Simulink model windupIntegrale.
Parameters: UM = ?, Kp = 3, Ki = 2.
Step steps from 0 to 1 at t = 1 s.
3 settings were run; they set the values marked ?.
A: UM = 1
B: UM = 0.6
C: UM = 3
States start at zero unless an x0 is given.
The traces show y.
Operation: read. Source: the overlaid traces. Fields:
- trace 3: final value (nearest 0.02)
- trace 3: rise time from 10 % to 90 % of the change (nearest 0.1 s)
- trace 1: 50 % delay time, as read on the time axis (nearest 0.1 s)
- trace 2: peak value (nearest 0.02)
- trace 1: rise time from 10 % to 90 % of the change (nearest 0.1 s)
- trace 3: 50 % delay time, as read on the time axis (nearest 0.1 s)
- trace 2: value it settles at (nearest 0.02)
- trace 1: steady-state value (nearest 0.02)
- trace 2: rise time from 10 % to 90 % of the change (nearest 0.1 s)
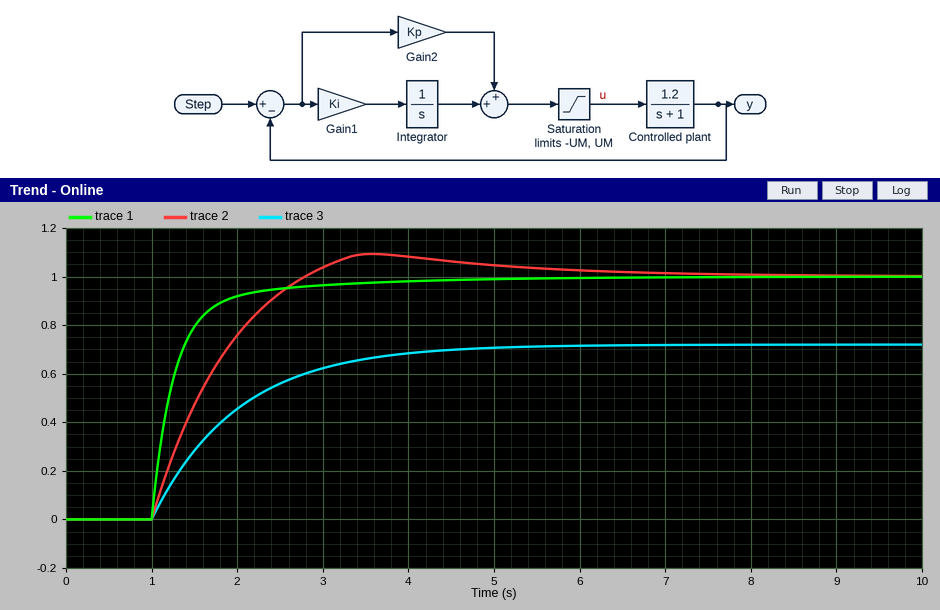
0.72
2.2 s
1.2 s
1.10
0.8 s
1.7 s
1.00
1.00
1.3 s
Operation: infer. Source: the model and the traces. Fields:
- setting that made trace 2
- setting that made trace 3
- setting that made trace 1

A
B
C
